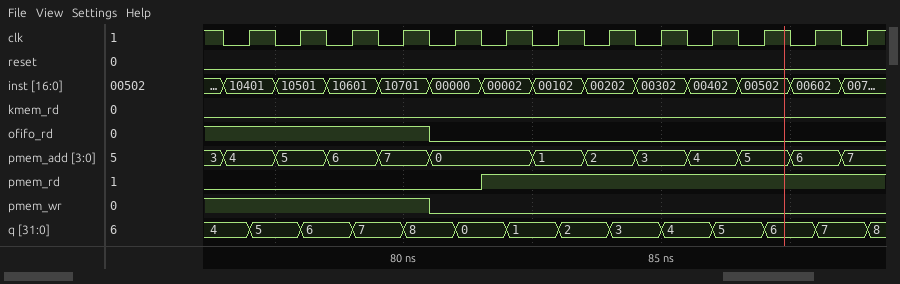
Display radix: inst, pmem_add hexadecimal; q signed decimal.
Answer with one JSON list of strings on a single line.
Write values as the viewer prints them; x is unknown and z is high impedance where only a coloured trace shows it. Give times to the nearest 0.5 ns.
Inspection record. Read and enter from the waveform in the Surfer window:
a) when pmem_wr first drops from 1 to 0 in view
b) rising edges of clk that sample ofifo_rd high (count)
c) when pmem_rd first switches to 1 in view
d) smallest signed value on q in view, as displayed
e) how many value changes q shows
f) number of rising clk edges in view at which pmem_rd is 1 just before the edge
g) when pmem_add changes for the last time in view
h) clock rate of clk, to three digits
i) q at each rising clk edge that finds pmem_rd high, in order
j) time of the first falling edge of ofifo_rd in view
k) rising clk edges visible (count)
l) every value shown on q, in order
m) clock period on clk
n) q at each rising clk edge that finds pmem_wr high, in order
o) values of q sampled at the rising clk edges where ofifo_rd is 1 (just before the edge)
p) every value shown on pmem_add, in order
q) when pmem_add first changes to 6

["80.5 ns", "4", "81.5 ns", "0", "13", "8", "88.5 ns", "1.00 GHz", "0, 1, 2, 3, 4, 5, 6, 7", "80.5 ns", "13", "4, 5, 6, 7, 8, 0, 1, 2, 3, 4, 5, 6, 7, 8", "1 ns", "4, 5, 6, 7", "4, 5, 6, 7", "3, 4, 5, 6, 7, 0, 1, 2, 3, 4, 5, 6, 7", "78.5 ns"]
